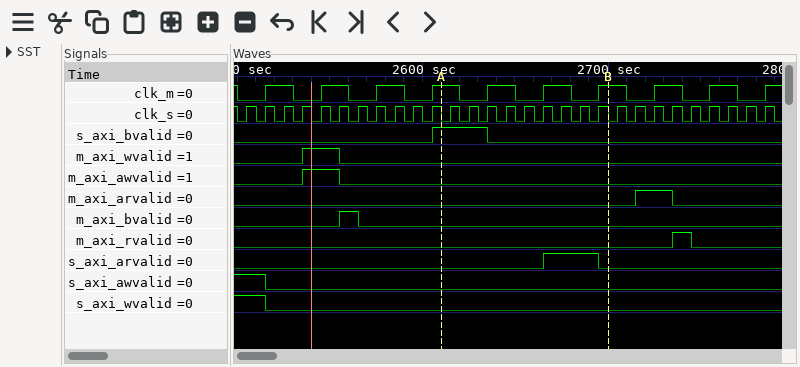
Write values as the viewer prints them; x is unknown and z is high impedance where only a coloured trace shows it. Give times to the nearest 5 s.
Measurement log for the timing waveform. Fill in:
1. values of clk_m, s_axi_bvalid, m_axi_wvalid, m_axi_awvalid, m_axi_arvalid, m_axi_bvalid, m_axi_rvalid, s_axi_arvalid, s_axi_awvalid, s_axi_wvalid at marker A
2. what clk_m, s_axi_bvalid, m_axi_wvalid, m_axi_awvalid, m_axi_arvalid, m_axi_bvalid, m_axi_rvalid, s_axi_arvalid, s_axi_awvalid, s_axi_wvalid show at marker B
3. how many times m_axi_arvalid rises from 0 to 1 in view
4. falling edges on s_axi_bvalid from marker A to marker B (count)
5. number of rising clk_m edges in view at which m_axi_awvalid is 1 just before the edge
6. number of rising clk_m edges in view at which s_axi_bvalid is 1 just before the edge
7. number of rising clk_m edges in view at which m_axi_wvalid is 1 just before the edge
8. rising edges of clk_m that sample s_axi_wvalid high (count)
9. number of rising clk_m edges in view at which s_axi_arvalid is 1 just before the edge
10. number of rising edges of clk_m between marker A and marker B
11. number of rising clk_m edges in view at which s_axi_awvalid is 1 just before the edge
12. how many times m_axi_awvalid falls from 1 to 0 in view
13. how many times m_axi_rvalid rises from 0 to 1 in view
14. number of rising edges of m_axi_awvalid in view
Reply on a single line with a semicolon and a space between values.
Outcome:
clk_m=1, s_axi_bvalid=1, m_axi_wvalid=0, m_axi_awvalid=0, m_axi_arvalid=0, m_axi_bvalid=0, m_axi_rvalid=0, s_axi_arvalid=0, s_axi_awvalid=0, s_axi_wvalid=0; clk_m=1, s_axi_bvalid=0, m_axi_wvalid=0, m_axi_awvalid=0, m_axi_arvalid=0, m_axi_bvalid=0, m_axi_rvalid=0, s_axi_arvalid=0, s_axi_awvalid=0, s_axi_wvalid=0; 1; 1; 1; 1; 1; 1; 1; 3; 1; 1; 1; 1
